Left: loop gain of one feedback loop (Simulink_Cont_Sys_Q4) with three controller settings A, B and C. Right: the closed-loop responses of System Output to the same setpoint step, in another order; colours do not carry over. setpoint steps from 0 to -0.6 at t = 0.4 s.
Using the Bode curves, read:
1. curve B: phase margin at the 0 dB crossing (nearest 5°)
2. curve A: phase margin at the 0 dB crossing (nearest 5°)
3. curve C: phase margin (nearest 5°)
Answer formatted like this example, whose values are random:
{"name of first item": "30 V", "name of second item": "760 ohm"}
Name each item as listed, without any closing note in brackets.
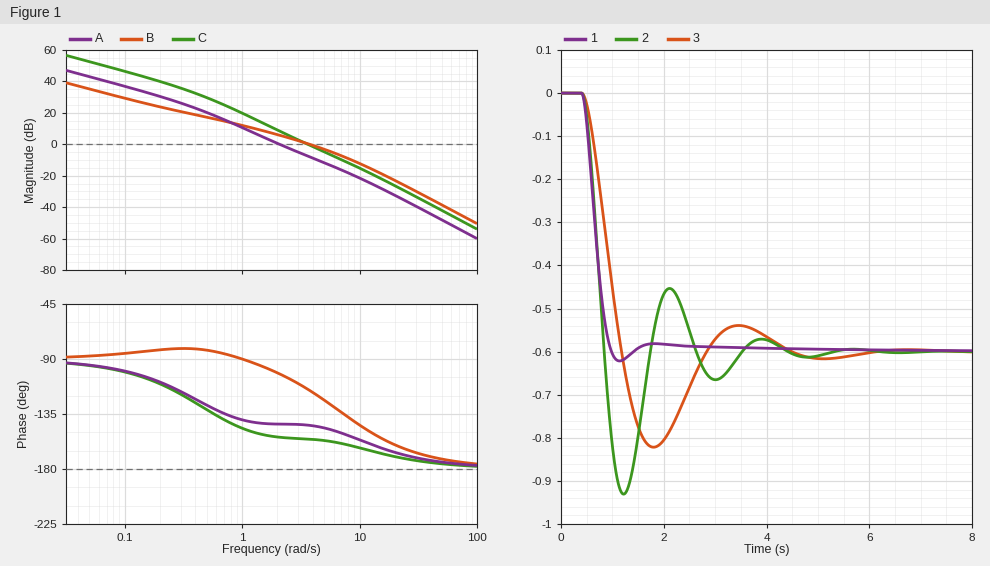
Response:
{"curve B: phase margin at the 0 dB crossing": "65°", "curve A: phase margin at the 0 dB crossing": "35°", "curve C: phase margin": "25°"}
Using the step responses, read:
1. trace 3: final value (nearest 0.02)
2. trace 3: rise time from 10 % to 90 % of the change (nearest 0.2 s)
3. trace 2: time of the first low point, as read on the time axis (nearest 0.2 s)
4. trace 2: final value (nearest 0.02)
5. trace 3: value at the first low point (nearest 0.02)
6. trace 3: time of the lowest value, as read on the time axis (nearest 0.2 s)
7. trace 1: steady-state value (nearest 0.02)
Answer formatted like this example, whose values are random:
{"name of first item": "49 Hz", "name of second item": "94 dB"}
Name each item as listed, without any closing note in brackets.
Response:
{"trace 3: final value": "-0.60", "trace 3: rise time from 10 % to 90 % of the change": "0.6 s", "trace 2: time of the first low point, as read on the time axis": "1.2 s", "trace 2: final value": "-0.60", "trace 3: value at the first low point": "-0.82", "trace 3: time of the lowest value, as read on the time axis": "1.8 s", "trace 1: steady-state value": "-0.60"}
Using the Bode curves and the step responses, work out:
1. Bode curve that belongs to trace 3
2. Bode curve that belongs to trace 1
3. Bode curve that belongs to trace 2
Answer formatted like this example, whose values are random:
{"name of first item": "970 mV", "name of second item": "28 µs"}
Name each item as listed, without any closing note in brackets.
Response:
{"Bode curve that belongs to trace 3": "A", "Bode curve that belongs to trace 1": "B", "Bode curve that belongs to trace 2": "C"}
